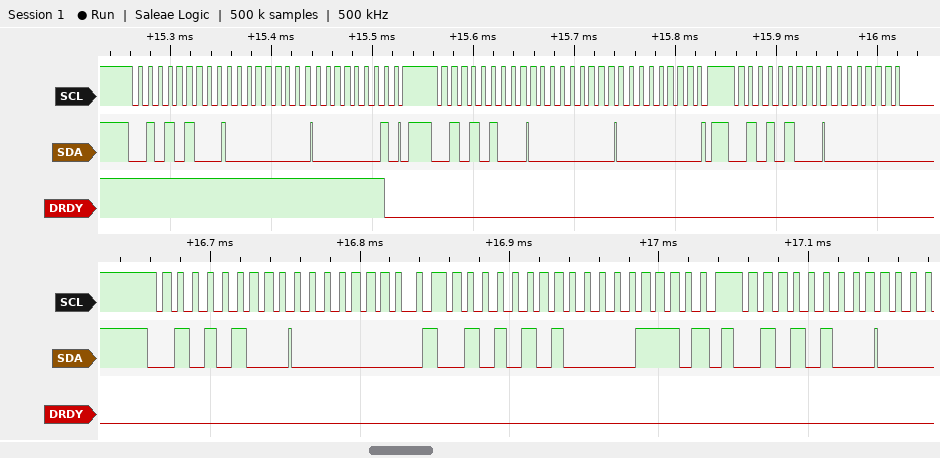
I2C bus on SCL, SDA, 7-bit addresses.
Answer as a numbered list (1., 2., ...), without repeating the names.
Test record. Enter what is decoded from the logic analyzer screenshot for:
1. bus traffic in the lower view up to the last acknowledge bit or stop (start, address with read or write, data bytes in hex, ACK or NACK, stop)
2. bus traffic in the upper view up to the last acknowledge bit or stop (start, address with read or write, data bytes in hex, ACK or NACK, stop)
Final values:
1. start, address 2A write ACK, 00 ACK, repeated start, address 2A read ACK, 0E NACK, stop, start, address 2A write ACK
2. start, address 2A write ACK, 00 ACK, 01 ACK, stop, start, address 2A write ACK, 00 ACK, 00 ACK, stop, start, address 2A write ACK
